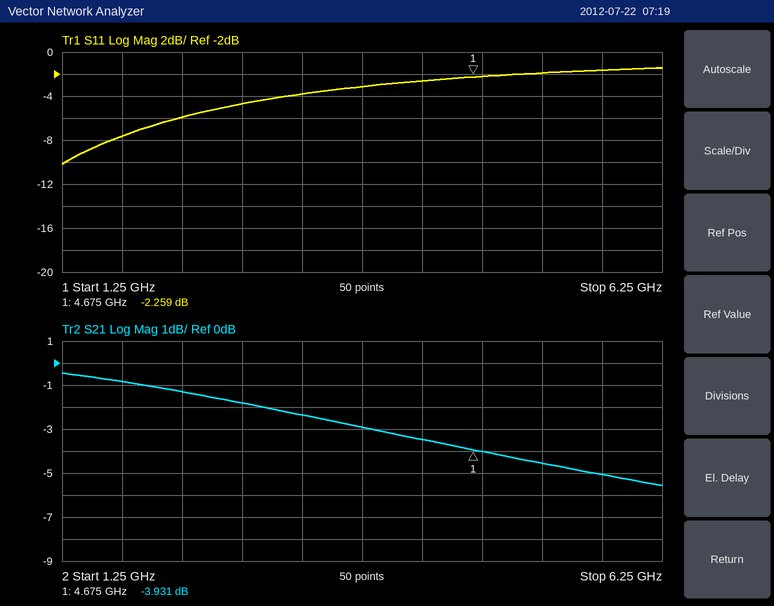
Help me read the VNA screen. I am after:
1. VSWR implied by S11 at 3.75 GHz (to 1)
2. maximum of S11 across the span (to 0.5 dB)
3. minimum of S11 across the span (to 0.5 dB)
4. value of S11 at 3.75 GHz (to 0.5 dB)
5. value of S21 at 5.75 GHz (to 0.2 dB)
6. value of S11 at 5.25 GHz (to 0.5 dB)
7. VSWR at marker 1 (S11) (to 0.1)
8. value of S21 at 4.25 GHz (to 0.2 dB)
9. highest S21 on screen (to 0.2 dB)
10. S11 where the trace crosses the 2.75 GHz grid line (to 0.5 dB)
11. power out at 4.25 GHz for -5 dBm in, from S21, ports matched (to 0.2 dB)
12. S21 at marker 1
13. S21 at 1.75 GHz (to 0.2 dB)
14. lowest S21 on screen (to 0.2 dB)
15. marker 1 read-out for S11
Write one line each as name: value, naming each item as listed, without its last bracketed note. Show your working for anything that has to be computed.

VSWR implied by S11 at 3.75 GHz: |Γ| = 10^(-3/20) = 0.7079; VSWR = (1 + 0.7079)/(1 − 0.7079) ≈ 6
maximum of S11 across the span: -1.5 dB
minimum of S11 across the span: -10.0 dB
value of S11 at 3.75 GHz: -3.0 dB
value of S21 at 5.75 GHz: -5.0 dB
value of S11 at 5.25 GHz: -2.0 dB
VSWR at marker 1 (S11): (1 + 0.7710)/(1 − 0.7710) ≈ 7.7
value of S21 at 4.25 GHz: -3.4 dB
highest S21 on screen: -0.4 dB
S11 where the trace crosses the 2.75 GHz grid line: -4.5 dB
power out at 4.25 GHz for -5 dBm in, from S21, ports matched: -5 dBm + (-3.4 dB) = -8.4 dBm
S21 at marker 1: -3.931 dB
S21 at 1.75 GHz: -0.8 dB
lowest S21 on screen: -5.6 dB
marker 1 read-out for S11: -2.259 dB
